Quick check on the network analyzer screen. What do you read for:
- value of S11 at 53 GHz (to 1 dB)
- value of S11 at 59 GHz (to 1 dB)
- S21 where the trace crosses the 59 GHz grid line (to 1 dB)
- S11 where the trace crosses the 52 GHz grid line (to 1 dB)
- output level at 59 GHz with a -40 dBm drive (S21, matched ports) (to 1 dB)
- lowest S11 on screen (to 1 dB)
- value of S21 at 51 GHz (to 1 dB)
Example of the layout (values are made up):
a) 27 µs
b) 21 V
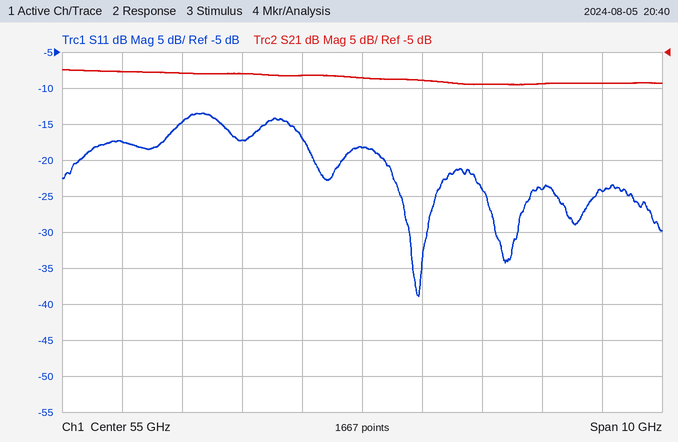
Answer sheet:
a) -17 dB
b) -24 dB
c) -9 dB
d) -15 dB
e) -49 dBm
f) -39 dB
g) -8 dB
